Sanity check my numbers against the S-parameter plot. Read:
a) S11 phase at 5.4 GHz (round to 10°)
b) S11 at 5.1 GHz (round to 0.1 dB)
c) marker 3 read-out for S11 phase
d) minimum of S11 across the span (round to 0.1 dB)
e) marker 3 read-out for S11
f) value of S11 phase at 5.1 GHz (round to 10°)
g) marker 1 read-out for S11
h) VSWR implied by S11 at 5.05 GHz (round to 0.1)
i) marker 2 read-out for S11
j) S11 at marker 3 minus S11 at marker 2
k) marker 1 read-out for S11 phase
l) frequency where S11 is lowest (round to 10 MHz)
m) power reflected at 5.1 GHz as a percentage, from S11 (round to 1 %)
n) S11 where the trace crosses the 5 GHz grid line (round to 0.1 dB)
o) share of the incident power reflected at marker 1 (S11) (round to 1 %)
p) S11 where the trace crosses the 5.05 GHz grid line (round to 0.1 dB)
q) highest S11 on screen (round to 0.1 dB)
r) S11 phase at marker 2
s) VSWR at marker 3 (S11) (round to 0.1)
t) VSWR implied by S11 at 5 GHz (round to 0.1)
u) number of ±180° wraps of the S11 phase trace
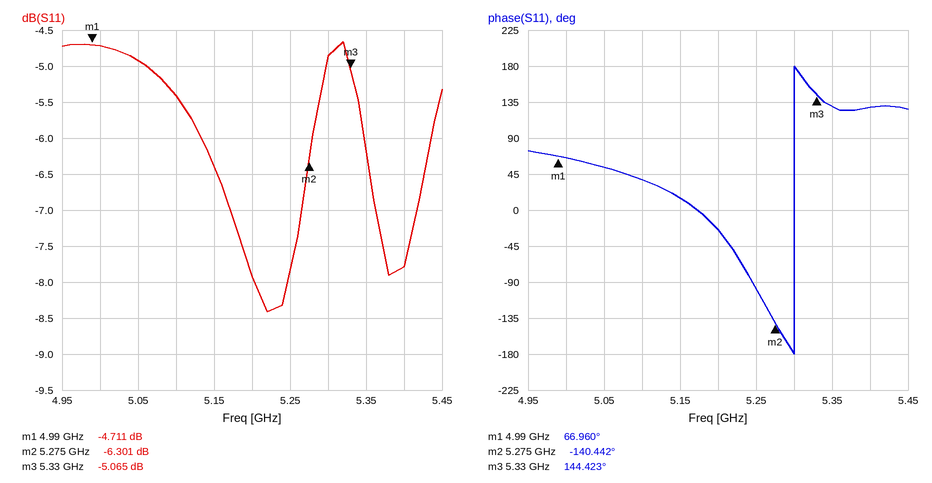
130°
-5.4 dB
144.423°
-8.4 dB
-5.065 dB
40°
-4.711 dB
3.6
-6.301 dB
1.236 dB
66.960°
5.22 GHz
29 %
-4.7 dB
34 %
-4.9 dB
-4.7 dB
-140.442°
3.5
3.8
1
